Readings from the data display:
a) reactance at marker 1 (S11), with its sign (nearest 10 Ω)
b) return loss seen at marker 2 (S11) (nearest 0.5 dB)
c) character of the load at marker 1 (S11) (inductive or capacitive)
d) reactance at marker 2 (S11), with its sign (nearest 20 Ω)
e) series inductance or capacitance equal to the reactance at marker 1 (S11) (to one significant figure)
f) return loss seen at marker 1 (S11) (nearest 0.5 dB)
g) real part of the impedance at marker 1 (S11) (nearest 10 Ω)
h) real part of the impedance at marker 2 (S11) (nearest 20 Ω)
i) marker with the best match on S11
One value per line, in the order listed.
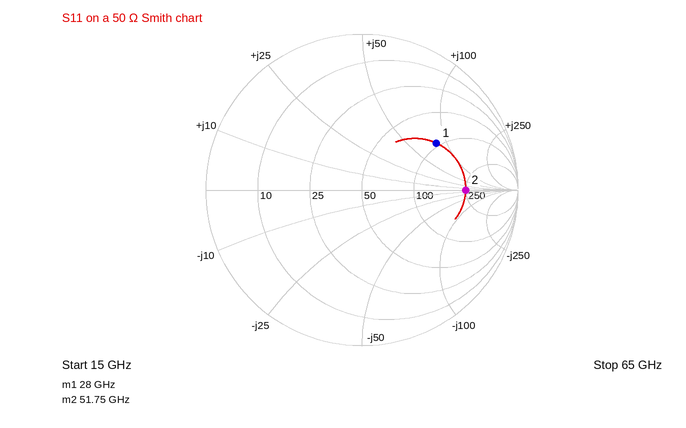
+80 Ω
3.5 dB
inductive
0 Ω
500 pH
5.0 dB
90 Ω
240 Ω
marker 1
